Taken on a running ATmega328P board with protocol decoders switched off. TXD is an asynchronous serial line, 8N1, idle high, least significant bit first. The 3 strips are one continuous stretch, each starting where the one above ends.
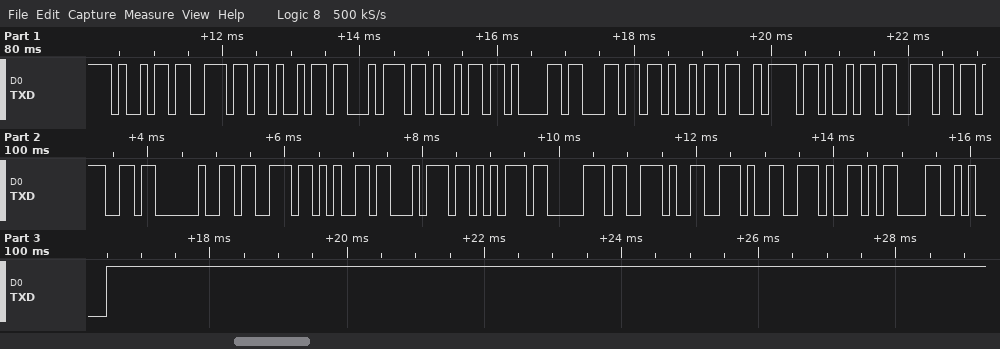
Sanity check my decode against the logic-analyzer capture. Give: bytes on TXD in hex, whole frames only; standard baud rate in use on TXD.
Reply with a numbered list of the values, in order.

1. 0x69 0x6E 0x69 0x74 0x69 0x61 0x6C 0x69 0x7A 0x69 0x6E 0x67 0x20 0x73 0x65 0x74 0x75 0x70 0x2E 0x2E 0x2E 0x0D 0x0A
2. 9600 baud
